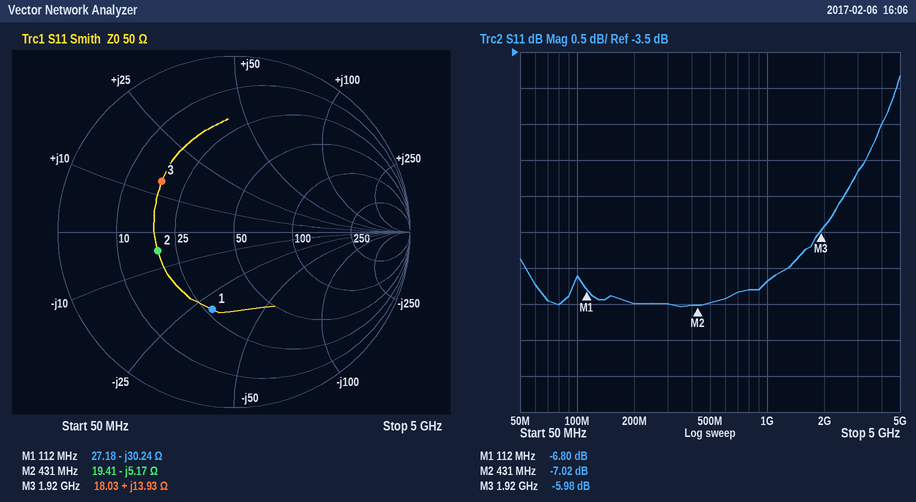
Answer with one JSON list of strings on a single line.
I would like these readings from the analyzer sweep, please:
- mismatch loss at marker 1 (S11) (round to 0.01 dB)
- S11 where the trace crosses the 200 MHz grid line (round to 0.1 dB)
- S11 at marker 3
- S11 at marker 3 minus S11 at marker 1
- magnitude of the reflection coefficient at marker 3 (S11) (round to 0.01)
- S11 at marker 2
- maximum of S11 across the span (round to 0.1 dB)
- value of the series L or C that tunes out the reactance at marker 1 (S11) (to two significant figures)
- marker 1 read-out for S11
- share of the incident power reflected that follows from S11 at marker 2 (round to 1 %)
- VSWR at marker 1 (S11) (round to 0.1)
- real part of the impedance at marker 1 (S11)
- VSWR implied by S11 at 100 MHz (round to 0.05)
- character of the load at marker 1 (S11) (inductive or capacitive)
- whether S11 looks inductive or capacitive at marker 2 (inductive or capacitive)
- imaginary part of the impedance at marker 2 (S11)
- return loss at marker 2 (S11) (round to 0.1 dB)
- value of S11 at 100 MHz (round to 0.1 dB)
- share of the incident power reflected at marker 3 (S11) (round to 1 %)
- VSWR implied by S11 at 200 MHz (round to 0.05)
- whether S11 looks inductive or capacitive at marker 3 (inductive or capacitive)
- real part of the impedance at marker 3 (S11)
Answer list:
["1.02 dB", "-7.0 dB", "-5.98 dB", "0.82 dB", "0.50", "-7.02 dB", "-3.8 dB", "43 nH", "-6.80 dB", "20 %", "2.7", "27.18 Ω", "2.75", "capacitive", "capacitive", "-5.17 Ω", "7.0 dB", "-6.6 dB", "25 %", "2.60", "inductive", "18.03 Ω"]
